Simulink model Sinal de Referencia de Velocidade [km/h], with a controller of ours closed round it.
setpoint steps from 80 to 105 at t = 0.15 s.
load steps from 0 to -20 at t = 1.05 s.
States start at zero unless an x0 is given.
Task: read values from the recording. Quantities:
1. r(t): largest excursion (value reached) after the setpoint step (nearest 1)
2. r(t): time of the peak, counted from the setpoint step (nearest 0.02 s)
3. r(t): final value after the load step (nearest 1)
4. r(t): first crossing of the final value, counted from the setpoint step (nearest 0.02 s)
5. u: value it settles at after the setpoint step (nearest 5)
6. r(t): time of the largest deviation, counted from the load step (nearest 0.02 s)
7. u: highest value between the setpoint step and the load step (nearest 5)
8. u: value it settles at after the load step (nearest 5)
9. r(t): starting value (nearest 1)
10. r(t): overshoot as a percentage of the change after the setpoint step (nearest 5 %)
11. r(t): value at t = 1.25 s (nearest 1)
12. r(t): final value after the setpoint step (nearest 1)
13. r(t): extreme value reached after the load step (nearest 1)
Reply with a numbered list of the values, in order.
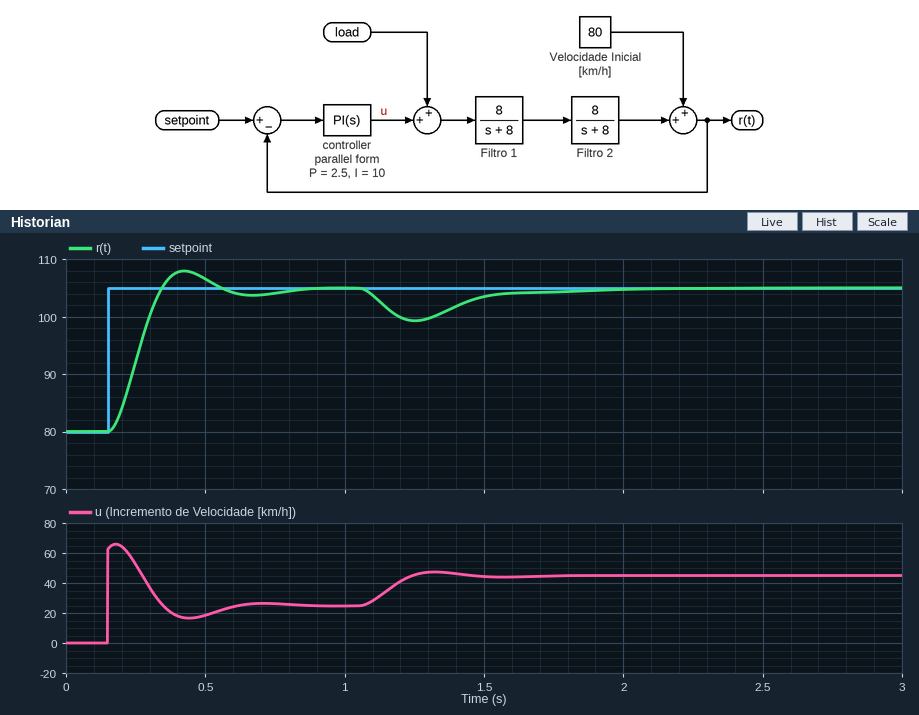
1. 108
2. 0.28 s
3. 105
4. 0.20 s
5. 25
6. 0.20 s
7. 65
8. 45
9. 80
10. 10 %
11. 99
12. 105
13. 99
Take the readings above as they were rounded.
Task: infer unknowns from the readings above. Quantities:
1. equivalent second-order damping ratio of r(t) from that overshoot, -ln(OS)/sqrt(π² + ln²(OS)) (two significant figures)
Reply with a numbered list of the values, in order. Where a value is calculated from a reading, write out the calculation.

1. ln(0.1) = -2.303; 2.303 / sqrt(9.870 + 5.302) = 0.59
